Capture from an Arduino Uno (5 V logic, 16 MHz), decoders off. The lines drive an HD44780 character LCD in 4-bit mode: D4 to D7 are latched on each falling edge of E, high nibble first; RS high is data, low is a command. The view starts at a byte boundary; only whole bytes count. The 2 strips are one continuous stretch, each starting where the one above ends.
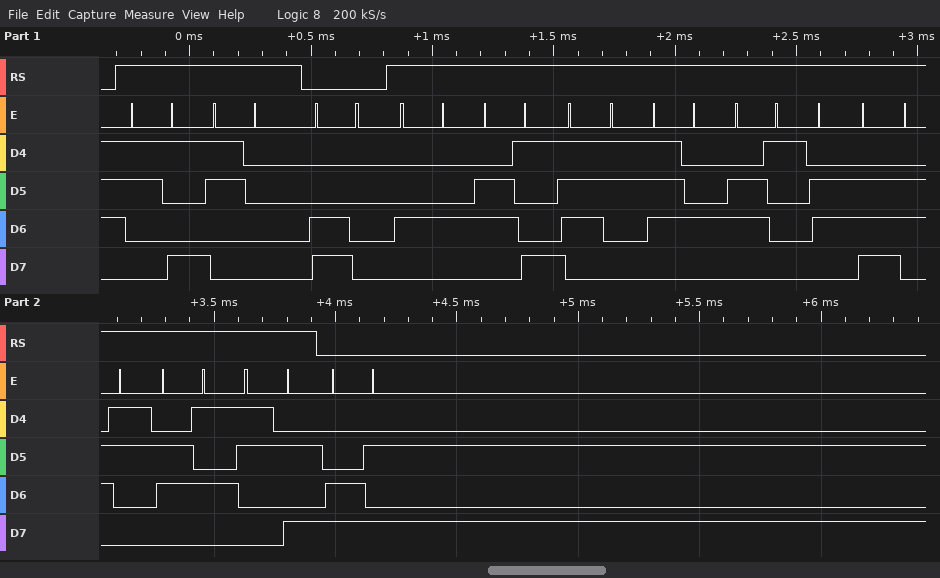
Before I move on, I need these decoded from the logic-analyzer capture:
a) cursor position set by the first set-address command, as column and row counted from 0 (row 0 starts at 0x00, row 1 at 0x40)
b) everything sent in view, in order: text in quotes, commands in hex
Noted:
column 0, row 1
"90" 0xC0 "Distance:" 0xCA
